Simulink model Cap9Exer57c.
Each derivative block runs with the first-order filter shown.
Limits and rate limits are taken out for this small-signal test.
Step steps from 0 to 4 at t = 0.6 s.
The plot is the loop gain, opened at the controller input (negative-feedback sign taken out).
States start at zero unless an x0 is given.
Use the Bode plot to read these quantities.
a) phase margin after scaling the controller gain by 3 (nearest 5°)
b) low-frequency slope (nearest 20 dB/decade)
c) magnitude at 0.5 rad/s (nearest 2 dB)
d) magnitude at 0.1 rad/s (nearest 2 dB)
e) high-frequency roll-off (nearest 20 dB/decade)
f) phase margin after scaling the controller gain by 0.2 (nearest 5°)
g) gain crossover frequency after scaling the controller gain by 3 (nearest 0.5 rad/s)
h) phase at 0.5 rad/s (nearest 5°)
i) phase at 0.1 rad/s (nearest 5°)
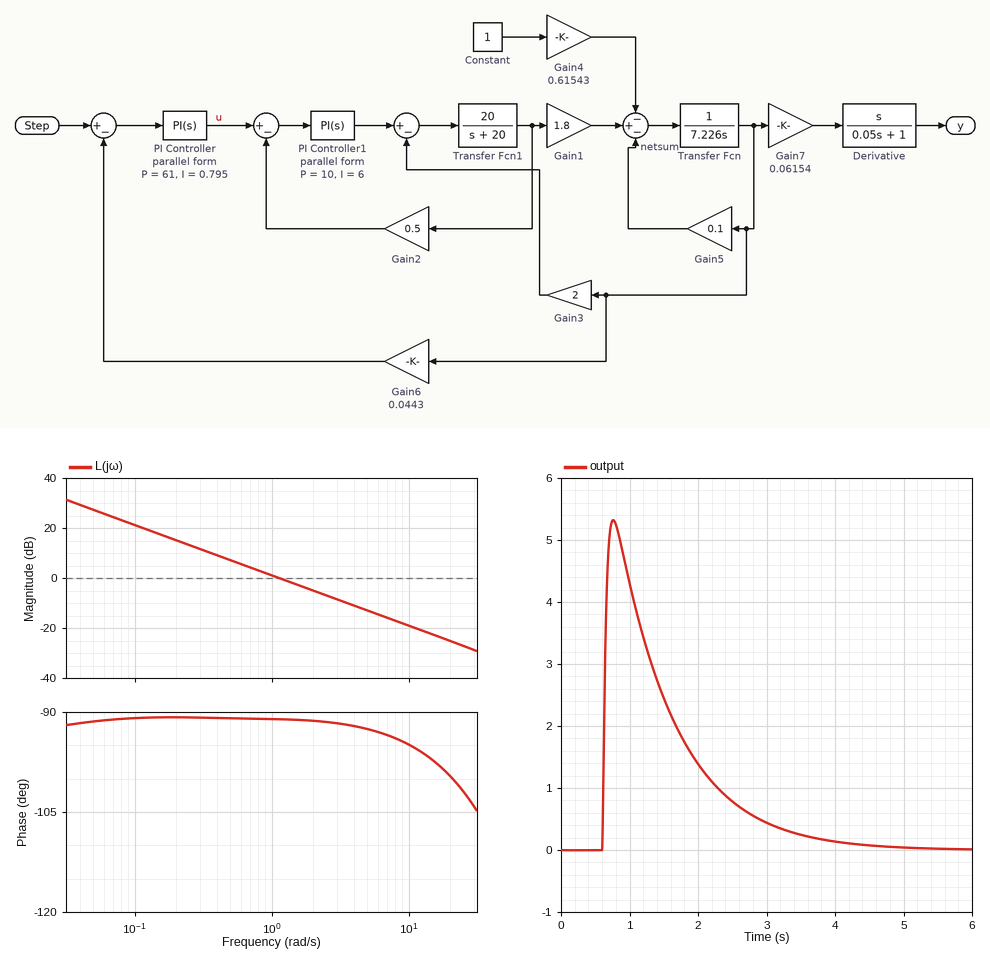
90°
-20 dB/decade
8 dB
22 dB
-20 dB/decade
90°
3.5 rad/s
-90°
-90°
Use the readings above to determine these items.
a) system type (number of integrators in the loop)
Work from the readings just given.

1
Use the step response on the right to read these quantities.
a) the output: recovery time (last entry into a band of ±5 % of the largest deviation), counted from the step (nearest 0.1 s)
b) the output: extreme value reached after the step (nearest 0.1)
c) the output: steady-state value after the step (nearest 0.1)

2.8 s
5.3
0.0
